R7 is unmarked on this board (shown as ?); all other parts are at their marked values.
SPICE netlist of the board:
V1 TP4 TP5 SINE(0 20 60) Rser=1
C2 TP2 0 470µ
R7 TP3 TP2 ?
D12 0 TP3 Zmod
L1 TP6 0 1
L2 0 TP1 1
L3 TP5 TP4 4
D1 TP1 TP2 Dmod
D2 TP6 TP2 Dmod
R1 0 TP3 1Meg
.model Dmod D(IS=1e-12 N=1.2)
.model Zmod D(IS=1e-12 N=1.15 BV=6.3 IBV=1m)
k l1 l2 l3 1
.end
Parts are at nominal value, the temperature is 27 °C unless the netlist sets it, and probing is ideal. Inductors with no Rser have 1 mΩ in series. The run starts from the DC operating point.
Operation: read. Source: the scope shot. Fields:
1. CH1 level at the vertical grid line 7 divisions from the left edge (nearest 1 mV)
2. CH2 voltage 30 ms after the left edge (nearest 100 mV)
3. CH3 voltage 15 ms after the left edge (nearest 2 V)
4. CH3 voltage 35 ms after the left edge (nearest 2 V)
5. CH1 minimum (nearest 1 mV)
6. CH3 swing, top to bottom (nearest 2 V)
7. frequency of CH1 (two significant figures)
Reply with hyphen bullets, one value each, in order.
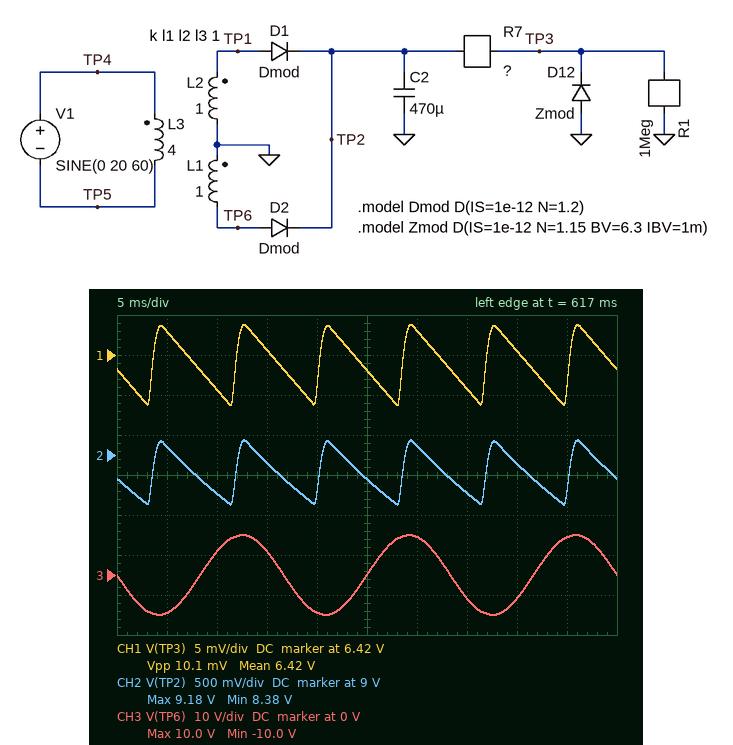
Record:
- 6.416 V
- 9.1 V
- 6 V
- -6 V
- 6.414 V
- 20 V
- 120 Hz
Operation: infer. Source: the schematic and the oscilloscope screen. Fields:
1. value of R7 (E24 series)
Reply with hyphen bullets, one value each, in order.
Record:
- 43 Ω
